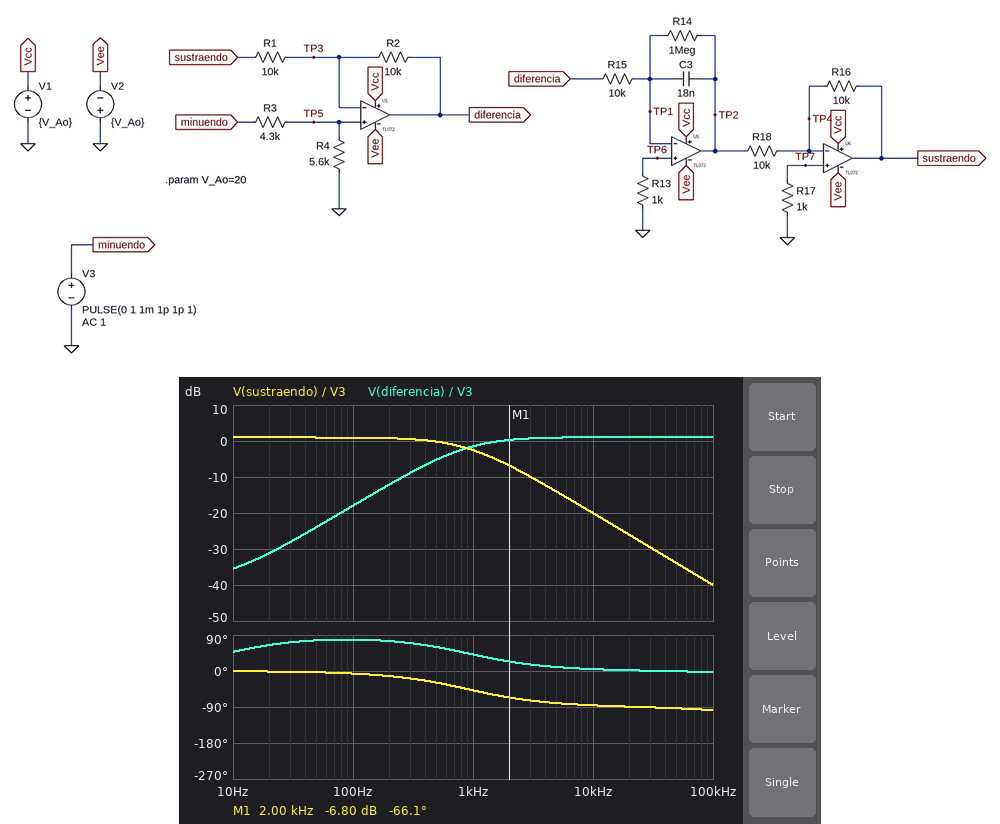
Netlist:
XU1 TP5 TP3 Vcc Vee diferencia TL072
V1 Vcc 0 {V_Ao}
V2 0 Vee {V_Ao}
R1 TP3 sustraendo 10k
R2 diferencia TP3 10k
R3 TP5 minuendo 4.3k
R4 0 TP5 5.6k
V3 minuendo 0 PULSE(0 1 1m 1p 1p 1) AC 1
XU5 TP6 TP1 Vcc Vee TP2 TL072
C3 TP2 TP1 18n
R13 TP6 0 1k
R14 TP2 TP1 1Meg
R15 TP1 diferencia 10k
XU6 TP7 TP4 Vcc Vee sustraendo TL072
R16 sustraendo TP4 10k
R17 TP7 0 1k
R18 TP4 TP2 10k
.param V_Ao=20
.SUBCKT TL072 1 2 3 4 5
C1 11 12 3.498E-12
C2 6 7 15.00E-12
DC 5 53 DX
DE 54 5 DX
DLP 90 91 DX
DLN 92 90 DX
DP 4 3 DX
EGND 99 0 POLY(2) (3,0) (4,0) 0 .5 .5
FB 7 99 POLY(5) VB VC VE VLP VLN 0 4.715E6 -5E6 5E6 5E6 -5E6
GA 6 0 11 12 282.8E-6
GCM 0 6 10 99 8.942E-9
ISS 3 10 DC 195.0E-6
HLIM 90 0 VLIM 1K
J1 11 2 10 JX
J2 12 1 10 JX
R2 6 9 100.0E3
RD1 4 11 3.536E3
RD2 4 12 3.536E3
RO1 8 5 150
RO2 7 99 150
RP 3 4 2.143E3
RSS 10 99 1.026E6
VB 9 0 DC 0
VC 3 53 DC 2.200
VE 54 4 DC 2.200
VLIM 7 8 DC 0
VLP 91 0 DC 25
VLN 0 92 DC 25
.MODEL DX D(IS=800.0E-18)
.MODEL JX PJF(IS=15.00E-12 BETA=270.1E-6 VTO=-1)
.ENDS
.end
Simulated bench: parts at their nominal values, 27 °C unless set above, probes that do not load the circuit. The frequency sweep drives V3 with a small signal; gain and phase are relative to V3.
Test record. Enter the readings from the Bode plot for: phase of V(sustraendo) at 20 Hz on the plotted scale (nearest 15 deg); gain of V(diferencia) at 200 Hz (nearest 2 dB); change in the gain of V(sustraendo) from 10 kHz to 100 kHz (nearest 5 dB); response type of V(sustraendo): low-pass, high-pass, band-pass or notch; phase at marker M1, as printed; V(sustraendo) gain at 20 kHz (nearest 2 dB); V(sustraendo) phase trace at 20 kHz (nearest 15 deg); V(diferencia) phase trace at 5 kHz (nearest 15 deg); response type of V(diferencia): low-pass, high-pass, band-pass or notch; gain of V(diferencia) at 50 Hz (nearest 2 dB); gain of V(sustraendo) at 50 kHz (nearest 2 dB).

0 deg
-12 dB
-20 dB
low-pass
-66.1 deg
-26 dB
-90 deg
15 deg
high-pass
-24 dB
-34 dB
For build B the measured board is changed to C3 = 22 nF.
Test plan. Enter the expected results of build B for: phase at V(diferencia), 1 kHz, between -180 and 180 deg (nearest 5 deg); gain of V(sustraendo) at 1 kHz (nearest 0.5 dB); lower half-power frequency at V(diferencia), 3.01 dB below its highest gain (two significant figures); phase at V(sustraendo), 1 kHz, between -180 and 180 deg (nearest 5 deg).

35 deg
-3.5 dB
730 Hz
-55 deg
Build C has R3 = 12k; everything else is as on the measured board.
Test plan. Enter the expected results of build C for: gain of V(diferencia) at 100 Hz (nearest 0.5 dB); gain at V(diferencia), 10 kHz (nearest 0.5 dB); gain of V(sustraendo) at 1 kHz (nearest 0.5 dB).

-23.0 dB
-4.0 dB
-7.5 dB
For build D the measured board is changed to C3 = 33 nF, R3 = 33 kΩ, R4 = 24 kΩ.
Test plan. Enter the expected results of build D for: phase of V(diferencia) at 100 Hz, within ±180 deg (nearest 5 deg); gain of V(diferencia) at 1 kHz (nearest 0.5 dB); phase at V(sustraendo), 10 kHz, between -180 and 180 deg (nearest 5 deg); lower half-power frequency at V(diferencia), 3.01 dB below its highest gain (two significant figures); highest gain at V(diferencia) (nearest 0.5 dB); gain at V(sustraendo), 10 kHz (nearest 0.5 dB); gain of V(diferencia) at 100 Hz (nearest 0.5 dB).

75 deg
-2.5 dB
-90 deg
490 Hz
-1.5 dB
-28.0 dB
-15.5 dB
